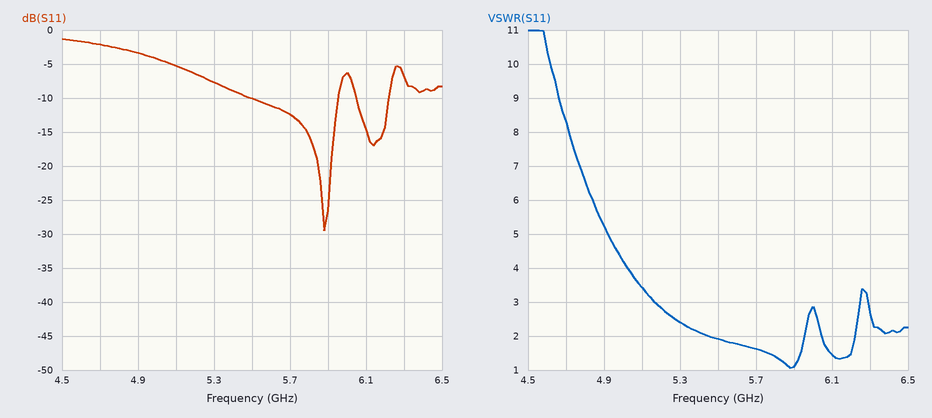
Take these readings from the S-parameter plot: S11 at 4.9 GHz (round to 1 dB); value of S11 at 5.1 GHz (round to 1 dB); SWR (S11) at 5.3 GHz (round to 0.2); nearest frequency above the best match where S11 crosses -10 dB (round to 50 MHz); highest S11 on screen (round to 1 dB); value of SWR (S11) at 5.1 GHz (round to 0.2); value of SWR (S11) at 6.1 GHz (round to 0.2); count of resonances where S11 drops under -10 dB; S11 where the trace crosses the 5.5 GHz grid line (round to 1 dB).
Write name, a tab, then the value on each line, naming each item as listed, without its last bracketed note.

S11 at 4.9 GHz	-3 dB
value of S11 at 5.1 GHz	-5 dB
SWR (S11) at 5.3 GHz	2.4
nearest frequency above the best match where S11 crosses -10 dB	5.95 GHz
highest S11 on screen	-1 dB
value of SWR (S11) at 5.1 GHz	3.4
value of SWR (S11) at 6.1 GHz	1.4
count of resonances where S11 drops under -10 dB	2
S11 where the trace crosses the 5.5 GHz grid line	-10 dB
